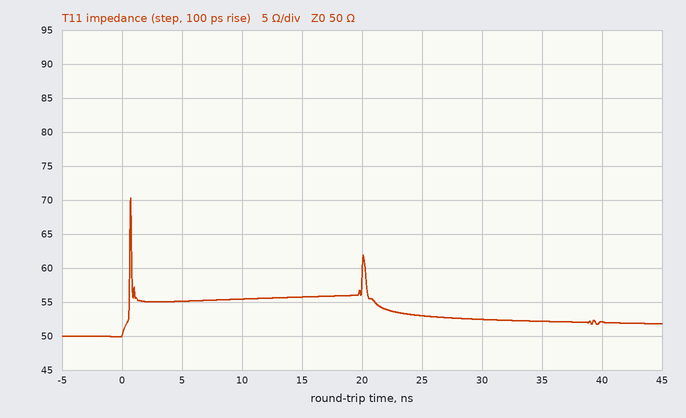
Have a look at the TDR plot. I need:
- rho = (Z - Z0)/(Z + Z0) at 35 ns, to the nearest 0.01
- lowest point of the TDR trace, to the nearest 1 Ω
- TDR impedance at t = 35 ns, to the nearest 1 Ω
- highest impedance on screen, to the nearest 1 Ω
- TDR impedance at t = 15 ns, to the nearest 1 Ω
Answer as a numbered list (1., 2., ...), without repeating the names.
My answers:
1. +0.02
2. 50 Ω
3. 52 Ω
4. 70 Ω
5. 56 Ω
